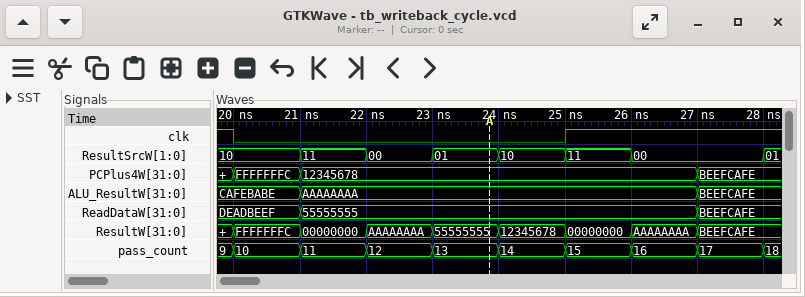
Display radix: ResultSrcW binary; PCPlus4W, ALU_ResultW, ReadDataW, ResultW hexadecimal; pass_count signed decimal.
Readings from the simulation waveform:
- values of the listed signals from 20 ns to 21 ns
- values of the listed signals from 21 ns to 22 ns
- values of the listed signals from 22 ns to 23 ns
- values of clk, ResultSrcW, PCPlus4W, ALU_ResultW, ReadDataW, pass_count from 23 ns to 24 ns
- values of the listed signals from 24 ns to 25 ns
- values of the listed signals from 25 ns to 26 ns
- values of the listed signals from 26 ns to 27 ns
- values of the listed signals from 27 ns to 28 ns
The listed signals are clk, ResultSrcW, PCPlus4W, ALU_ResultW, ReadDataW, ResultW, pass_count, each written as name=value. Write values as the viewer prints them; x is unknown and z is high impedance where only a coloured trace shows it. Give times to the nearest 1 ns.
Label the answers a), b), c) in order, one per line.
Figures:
a) clk=0, ResultSrcW=10, PCPlus4W=FFFFFFFC, ALU_ResultW=CAFEBABE, ReadDataW=DEADBEEF, ResultW=FFFFFFFC, pass_count=10
b) clk=0, ResultSrcW=11, PCPlus4W=12345678, ALU_ResultW=AAAAAAAA, ReadDataW=55555555, ResultW=00000000, pass_count=11
c) clk=0, ResultSrcW=00, PCPlus4W=12345678, ALU_ResultW=AAAAAAAA, ReadDataW=55555555, ResultW=AAAAAAAA, pass_count=12
d) clk=0, ResultSrcW=01, PCPlus4W=12345678, ALU_ResultW=AAAAAAAA, ReadDataW=55555555, pass_count=13
e) clk=0, ResultSrcW=10, PCPlus4W=12345678, ALU_ResultW=AAAAAAAA, ReadDataW=55555555, ResultW=12345678, pass_count=14
f) clk=1, ResultSrcW=11, PCPlus4W=12345678, ALU_ResultW=AAAAAAAA, ReadDataW=55555555, ResultW=00000000, pass_count=15
g) clk=1, ResultSrcW=00, PCPlus4W=12345678, ALU_ResultW=AAAAAAAA, ReadDataW=55555555, ResultW=AAAAAAAA, pass_count=16
h) clk=1, ResultSrcW=00, PCPlus4W=BEEFCAFE, ALU_ResultW=BEEFCAFE, ReadDataW=BEEFCAFE, ResultW=BEEFCAFE, pass_count=17
